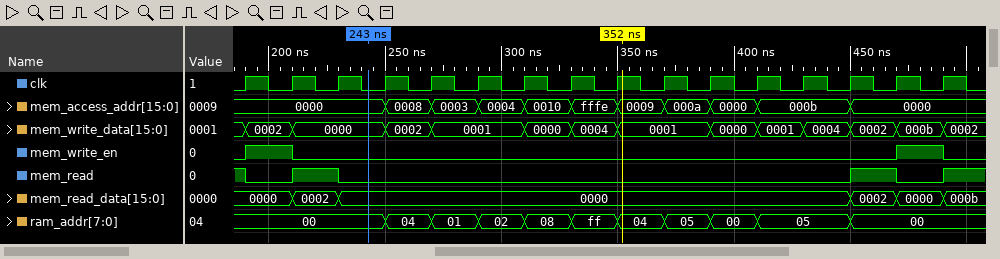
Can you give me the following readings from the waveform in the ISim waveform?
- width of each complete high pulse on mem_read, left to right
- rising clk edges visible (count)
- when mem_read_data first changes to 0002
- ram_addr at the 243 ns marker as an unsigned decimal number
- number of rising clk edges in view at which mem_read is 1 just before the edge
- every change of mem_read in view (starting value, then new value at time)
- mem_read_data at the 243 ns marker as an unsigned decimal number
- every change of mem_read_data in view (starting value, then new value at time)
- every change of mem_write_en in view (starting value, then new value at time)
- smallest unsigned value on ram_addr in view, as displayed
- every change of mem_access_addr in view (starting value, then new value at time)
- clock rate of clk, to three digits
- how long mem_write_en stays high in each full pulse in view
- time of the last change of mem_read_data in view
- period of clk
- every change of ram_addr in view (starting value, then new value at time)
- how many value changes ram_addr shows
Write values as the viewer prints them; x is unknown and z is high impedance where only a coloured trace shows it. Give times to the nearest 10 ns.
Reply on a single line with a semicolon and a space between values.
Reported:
20 ns, 20 ns; 16; 210 ns; 0; 3; 1, 0 at 190 ns, 1 at 210 ns, 0 at 230 ns, 1 at 450 ns, 0 at 470 ns, 1 at 490 ns; 0; 0000, 0002 at 210 ns, 0000 at 230 ns, 0002 at 450 ns, 0000 at 470 ns, 000b at 490 ns; 0, 1 at 190 ns, 0 at 210 ns, 1 at 470 ns, 0 at 490 ns; 00; 0000, 0008 at 250 ns, 0003 at 270 ns, 0004 at 290 ns, 0010 at 310 ns, fffe at 330 ns, 0009 at 350 ns, 000a at 370 ns, 0000 at 390 ns, 000b at 410 ns, 0000 at 450 ns; 50.0 MHz; 20 ns, 20 ns; 490 ns; 20 ns; 00, 04 at 250 ns, 01 at 270 ns, 02 at 290 ns, 08 at 310 ns, ff at 330 ns, 04 at 350 ns, 05 at 370 ns, 00 at 390 ns, 05 at 410 ns, 00 at 450 ns; 10
